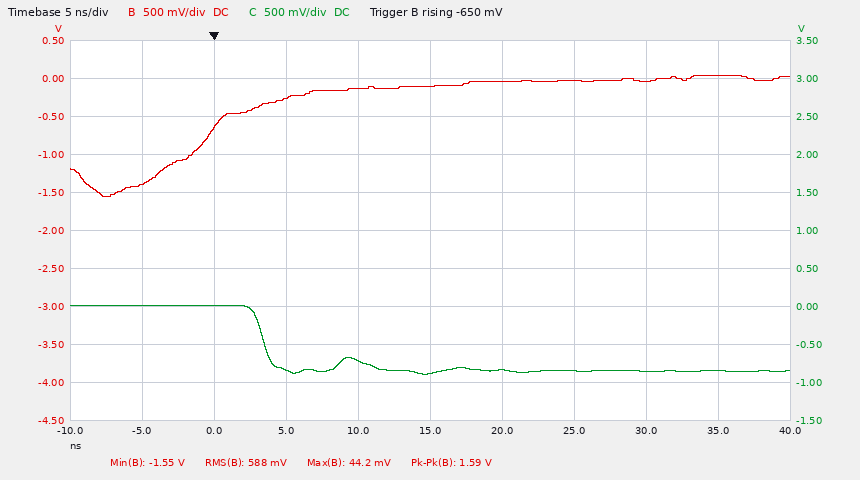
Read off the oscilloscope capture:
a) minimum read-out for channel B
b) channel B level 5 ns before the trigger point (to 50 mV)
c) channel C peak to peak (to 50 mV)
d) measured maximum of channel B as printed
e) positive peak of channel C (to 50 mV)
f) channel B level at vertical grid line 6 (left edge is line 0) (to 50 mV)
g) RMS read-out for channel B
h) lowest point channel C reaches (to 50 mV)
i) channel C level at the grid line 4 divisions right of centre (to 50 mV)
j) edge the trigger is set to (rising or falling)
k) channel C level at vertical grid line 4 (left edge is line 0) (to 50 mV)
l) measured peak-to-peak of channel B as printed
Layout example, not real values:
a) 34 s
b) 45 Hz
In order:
a) -1.55 V
b) -1.40 V
c) 900 mV
d) 44.2 mV
e) 0 mV
f) -50 mV
g) 588 mV
h) -900 mV
i) -850 mV
j) rising
k) -700 mV
l) 1.59 V
